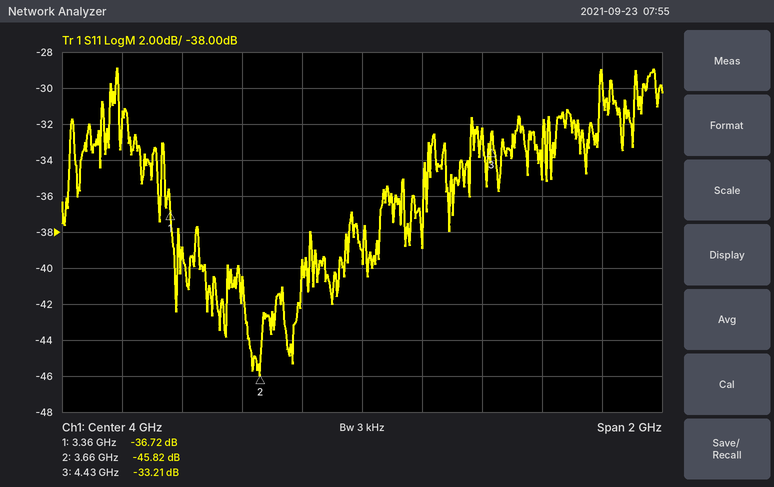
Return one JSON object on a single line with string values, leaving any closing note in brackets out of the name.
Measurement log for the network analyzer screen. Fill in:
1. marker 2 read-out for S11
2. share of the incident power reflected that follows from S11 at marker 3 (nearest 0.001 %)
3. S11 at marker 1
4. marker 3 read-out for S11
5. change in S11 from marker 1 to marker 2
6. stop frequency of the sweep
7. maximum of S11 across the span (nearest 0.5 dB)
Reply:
{"marker 2 read-out for S11": "-45.82 dB", "share of the incident power reflected that follows from S11 at marker 3": "0.048 %", "S11 at marker 1": "-36.72 dB", "marker 3 read-out for S11": "-33.21 dB", "change in S11 from marker 1 to marker 2": "-9.10 dB", "stop frequency of the sweep": "5 GHz", "maximum of S11 across the span": "-29.0 dB"}
